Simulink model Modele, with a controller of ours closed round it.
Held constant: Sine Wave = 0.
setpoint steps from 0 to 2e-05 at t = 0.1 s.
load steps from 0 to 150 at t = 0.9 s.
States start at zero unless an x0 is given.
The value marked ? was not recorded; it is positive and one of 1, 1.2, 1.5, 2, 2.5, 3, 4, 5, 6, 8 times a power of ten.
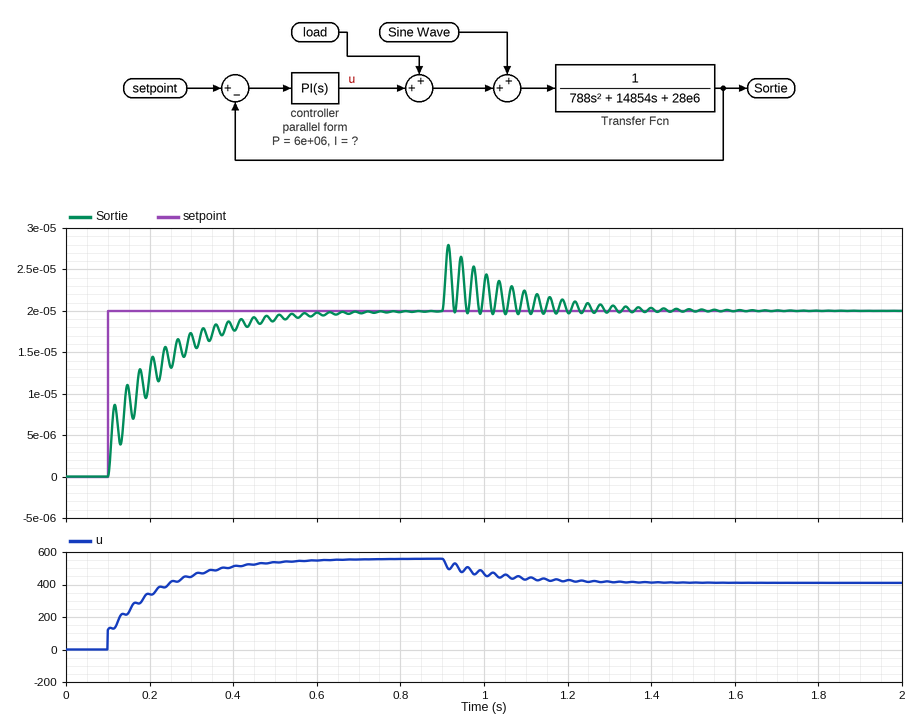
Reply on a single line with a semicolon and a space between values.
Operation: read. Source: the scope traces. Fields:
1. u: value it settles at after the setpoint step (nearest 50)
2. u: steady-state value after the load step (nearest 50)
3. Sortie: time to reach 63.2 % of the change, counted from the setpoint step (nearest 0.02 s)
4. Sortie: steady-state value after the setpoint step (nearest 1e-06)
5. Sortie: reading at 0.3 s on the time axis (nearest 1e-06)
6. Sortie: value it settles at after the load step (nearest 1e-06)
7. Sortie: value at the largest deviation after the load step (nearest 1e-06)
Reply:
550; 400; 0.08 s; 0.000020; 0.000017; 0.000020; 0.000028
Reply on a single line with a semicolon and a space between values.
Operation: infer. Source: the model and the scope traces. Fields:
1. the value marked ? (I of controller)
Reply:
2.5e+08
